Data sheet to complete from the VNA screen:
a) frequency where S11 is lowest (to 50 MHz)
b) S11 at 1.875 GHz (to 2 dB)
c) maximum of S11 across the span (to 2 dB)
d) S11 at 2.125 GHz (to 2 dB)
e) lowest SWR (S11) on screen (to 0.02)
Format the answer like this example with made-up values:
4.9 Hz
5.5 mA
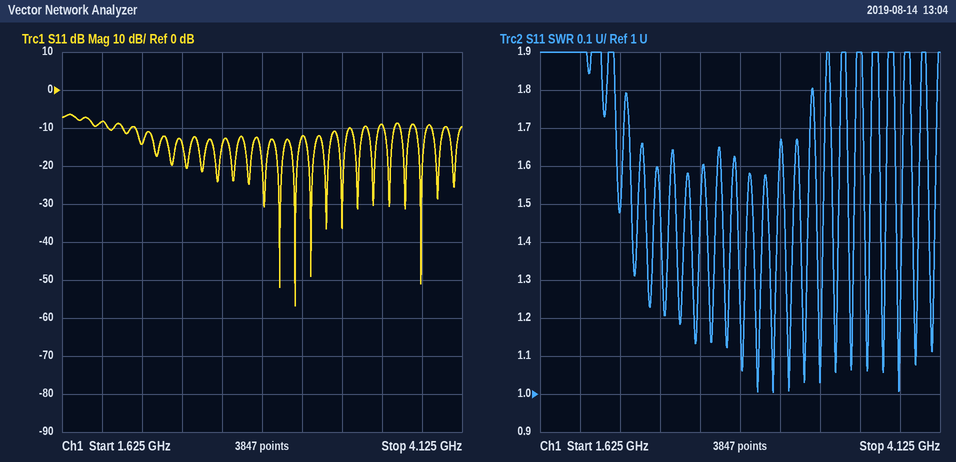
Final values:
3.10 GHz
-8 dB
-6 dB
-14 dB
1.00
